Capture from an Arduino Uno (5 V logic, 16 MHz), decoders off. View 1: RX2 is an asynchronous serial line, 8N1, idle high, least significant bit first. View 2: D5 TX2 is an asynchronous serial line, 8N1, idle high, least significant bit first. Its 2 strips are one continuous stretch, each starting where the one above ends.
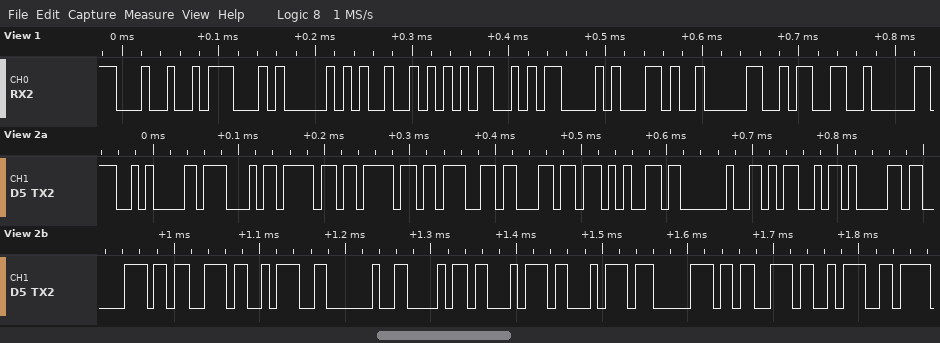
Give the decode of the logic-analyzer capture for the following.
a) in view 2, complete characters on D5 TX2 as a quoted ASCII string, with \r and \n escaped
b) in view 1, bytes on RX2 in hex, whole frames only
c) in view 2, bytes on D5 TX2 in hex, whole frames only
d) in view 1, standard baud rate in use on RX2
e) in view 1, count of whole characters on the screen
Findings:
"\nGoogle Maps: https:"
24 47 50 52 4D 43 2C 30 33
0A 47 6F 6F 67 6C 65 20 4D 61 70 73 3A 20 68 74 74 70 73 3A
115200 baud
9
